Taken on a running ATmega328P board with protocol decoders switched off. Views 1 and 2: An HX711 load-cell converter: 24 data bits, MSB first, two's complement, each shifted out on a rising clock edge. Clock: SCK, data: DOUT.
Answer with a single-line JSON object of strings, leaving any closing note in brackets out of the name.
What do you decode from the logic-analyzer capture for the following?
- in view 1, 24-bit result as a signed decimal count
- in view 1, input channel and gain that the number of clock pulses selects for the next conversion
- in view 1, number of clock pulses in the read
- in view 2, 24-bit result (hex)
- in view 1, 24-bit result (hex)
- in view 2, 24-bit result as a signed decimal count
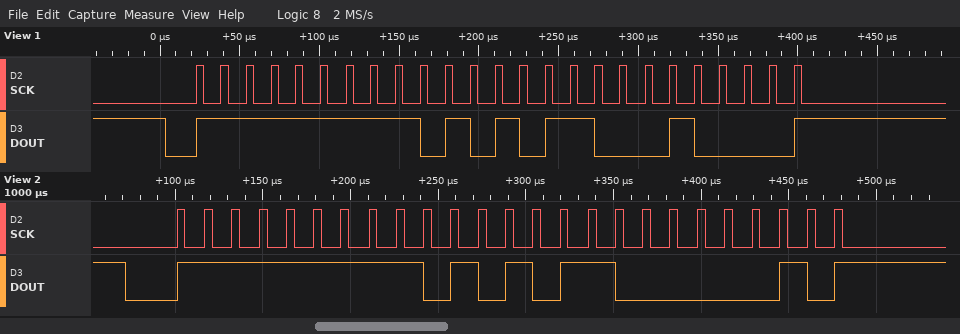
{"in view 1, 24-bit result as a signed decimal count": "-21744", "in view 1, input channel and gain that the number of clock pulses selects for the next conversion": "channel A, gain 128", "in view 1, number of clock pulses in the read": "25", "in view 2, 24-bit result": "0xFFAB02", "in view 1, 24-bit result": "0xFFAB10", "in view 2, 24-bit result as a signed decimal count": "-21758"}
